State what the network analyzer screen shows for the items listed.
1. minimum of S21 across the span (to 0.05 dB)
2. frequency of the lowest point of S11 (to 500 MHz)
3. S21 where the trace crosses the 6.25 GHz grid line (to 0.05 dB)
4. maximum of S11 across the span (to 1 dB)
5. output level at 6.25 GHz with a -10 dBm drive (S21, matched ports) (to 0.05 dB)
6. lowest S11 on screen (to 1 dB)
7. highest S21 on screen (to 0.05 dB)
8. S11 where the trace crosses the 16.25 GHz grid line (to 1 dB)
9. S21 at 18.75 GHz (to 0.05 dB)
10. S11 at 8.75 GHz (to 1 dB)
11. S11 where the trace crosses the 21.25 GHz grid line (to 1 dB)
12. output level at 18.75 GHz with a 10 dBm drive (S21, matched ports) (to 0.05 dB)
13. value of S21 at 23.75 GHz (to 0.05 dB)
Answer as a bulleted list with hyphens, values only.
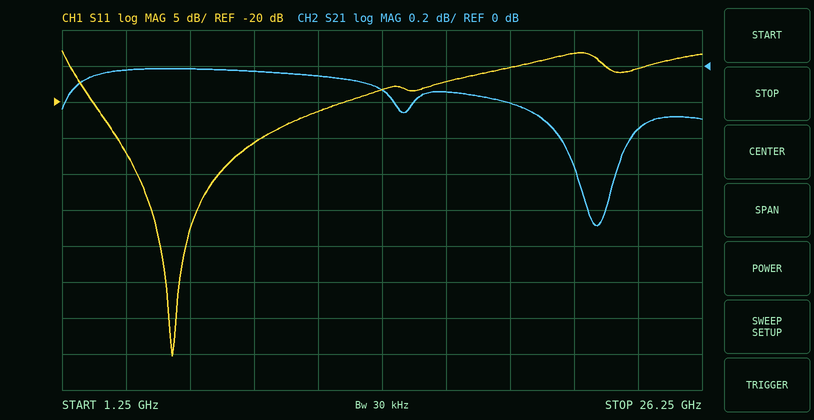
- -0.90 dB
- 5.5 GHz
- 0.00 dB
- -13 dB
- -10.00 dBm
- -55 dB
- 0.00 dB
- -17 dB
- -0.20 dB
- -26 dB
- -13 dB
- 9.80 dBm
- -0.35 dB
